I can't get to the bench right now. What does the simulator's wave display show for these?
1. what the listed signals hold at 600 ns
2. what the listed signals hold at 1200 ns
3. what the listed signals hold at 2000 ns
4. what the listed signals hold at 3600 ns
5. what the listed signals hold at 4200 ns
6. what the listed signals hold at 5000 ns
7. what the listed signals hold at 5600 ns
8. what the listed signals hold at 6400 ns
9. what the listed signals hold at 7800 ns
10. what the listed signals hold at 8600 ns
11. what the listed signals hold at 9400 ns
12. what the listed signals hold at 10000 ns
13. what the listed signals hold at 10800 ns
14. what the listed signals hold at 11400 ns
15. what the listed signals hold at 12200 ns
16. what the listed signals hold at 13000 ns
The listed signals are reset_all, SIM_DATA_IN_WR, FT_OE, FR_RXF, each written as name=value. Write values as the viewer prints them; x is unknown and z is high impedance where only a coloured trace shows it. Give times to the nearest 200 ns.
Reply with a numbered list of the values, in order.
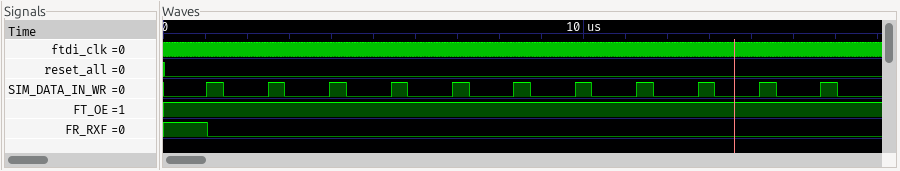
1. reset_all=0, SIM_DATA_IN_WR=0, FT_OE=1, FR_RXF=1
2. reset_all=0, SIM_DATA_IN_WR=1, FT_OE=1, FR_RXF=0
3. reset_all=0, SIM_DATA_IN_WR=0, FT_OE=1, FR_RXF=0
4. reset_all=0, SIM_DATA_IN_WR=0, FT_OE=1, FR_RXF=0
5. reset_all=0, SIM_DATA_IN_WR=1, FT_OE=1, FR_RXF=0
6. reset_all=0, SIM_DATA_IN_WR=0, FT_OE=1, FR_RXF=0
7. reset_all=0, SIM_DATA_IN_WR=1, FT_OE=1, FR_RXF=0
8. reset_all=0, SIM_DATA_IN_WR=0, FT_OE=1, FR_RXF=0
9. reset_all=0, SIM_DATA_IN_WR=0, FT_OE=1, FR_RXF=0
10. reset_all=0, SIM_DATA_IN_WR=1, FT_OE=1, FR_RXF=0
11. reset_all=0, SIM_DATA_IN_WR=0, FT_OE=1, FR_RXF=0
12. reset_all=0, SIM_DATA_IN_WR=1, FT_OE=1, FR_RXF=0
13. reset_all=0, SIM_DATA_IN_WR=0, FT_OE=1, FR_RXF=0
14. reset_all=0, SIM_DATA_IN_WR=1, FT_OE=1, FR_RXF=0
15. reset_all=0, SIM_DATA_IN_WR=0, FT_OE=1, FR_RXF=0
16. reset_all=0, SIM_DATA_IN_WR=1, FT_OE=1, FR_RXF=0
